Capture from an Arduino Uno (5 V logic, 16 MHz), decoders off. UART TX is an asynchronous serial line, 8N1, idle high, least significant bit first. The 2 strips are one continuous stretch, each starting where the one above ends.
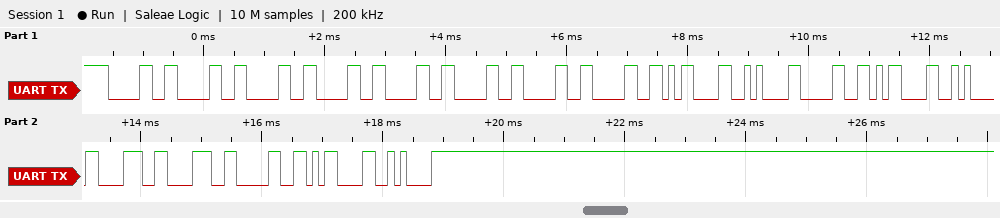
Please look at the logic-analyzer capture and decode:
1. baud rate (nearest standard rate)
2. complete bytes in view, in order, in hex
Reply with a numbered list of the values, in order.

1. 9600 baud
2. 30 30 30 30 30 30 30 30 0D 0A 30 0D 0A 38 38 30 0D 0A
